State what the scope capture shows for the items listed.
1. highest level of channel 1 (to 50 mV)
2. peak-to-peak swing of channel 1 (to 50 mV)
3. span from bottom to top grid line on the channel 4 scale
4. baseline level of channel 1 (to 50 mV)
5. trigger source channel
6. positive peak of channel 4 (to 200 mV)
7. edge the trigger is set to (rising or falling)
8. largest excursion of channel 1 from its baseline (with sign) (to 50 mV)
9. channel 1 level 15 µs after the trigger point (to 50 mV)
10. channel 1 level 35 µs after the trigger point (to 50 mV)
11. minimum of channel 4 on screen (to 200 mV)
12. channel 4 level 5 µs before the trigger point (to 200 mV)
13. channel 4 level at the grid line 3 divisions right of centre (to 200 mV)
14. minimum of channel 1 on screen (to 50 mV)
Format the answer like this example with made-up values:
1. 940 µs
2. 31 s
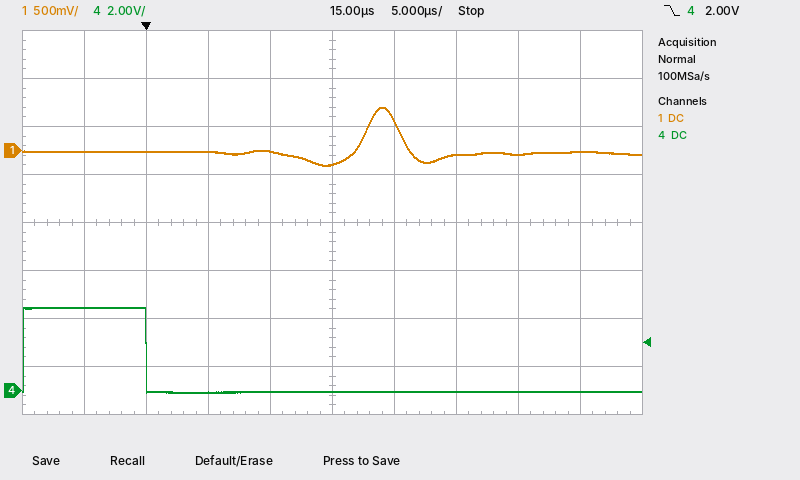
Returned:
1. 450 mV
2. 600 mV
3. 16 V
4. 0 mV
5. channel 4
6. 3.4 V
7. falling
8. +450 mV
9. -150 mV
10. 0 mV
11. 0.0 V
12. 3.4 V
13. 0.0 V
14. -150 mV
